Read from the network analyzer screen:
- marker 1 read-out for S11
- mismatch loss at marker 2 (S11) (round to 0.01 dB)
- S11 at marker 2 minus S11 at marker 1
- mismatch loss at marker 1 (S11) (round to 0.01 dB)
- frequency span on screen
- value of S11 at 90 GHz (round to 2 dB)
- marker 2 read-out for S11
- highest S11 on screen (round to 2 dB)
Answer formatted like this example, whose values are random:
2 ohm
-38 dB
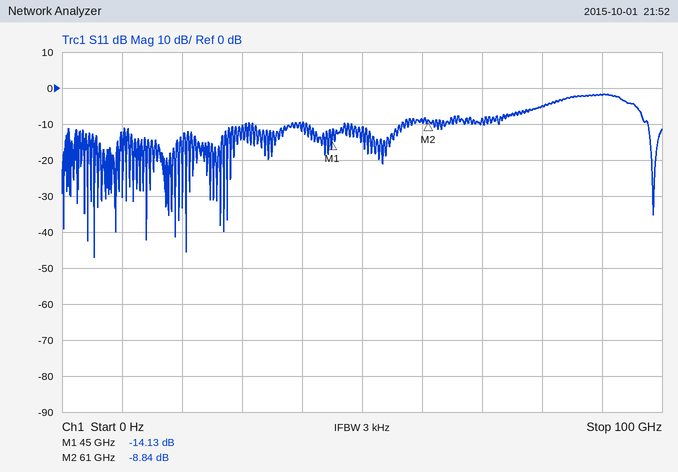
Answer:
-14.13 dB
0.61 dB
5.29 dB
0.17 dB
100 GHz
-2 dB
-8.84 dB
-2 dB
